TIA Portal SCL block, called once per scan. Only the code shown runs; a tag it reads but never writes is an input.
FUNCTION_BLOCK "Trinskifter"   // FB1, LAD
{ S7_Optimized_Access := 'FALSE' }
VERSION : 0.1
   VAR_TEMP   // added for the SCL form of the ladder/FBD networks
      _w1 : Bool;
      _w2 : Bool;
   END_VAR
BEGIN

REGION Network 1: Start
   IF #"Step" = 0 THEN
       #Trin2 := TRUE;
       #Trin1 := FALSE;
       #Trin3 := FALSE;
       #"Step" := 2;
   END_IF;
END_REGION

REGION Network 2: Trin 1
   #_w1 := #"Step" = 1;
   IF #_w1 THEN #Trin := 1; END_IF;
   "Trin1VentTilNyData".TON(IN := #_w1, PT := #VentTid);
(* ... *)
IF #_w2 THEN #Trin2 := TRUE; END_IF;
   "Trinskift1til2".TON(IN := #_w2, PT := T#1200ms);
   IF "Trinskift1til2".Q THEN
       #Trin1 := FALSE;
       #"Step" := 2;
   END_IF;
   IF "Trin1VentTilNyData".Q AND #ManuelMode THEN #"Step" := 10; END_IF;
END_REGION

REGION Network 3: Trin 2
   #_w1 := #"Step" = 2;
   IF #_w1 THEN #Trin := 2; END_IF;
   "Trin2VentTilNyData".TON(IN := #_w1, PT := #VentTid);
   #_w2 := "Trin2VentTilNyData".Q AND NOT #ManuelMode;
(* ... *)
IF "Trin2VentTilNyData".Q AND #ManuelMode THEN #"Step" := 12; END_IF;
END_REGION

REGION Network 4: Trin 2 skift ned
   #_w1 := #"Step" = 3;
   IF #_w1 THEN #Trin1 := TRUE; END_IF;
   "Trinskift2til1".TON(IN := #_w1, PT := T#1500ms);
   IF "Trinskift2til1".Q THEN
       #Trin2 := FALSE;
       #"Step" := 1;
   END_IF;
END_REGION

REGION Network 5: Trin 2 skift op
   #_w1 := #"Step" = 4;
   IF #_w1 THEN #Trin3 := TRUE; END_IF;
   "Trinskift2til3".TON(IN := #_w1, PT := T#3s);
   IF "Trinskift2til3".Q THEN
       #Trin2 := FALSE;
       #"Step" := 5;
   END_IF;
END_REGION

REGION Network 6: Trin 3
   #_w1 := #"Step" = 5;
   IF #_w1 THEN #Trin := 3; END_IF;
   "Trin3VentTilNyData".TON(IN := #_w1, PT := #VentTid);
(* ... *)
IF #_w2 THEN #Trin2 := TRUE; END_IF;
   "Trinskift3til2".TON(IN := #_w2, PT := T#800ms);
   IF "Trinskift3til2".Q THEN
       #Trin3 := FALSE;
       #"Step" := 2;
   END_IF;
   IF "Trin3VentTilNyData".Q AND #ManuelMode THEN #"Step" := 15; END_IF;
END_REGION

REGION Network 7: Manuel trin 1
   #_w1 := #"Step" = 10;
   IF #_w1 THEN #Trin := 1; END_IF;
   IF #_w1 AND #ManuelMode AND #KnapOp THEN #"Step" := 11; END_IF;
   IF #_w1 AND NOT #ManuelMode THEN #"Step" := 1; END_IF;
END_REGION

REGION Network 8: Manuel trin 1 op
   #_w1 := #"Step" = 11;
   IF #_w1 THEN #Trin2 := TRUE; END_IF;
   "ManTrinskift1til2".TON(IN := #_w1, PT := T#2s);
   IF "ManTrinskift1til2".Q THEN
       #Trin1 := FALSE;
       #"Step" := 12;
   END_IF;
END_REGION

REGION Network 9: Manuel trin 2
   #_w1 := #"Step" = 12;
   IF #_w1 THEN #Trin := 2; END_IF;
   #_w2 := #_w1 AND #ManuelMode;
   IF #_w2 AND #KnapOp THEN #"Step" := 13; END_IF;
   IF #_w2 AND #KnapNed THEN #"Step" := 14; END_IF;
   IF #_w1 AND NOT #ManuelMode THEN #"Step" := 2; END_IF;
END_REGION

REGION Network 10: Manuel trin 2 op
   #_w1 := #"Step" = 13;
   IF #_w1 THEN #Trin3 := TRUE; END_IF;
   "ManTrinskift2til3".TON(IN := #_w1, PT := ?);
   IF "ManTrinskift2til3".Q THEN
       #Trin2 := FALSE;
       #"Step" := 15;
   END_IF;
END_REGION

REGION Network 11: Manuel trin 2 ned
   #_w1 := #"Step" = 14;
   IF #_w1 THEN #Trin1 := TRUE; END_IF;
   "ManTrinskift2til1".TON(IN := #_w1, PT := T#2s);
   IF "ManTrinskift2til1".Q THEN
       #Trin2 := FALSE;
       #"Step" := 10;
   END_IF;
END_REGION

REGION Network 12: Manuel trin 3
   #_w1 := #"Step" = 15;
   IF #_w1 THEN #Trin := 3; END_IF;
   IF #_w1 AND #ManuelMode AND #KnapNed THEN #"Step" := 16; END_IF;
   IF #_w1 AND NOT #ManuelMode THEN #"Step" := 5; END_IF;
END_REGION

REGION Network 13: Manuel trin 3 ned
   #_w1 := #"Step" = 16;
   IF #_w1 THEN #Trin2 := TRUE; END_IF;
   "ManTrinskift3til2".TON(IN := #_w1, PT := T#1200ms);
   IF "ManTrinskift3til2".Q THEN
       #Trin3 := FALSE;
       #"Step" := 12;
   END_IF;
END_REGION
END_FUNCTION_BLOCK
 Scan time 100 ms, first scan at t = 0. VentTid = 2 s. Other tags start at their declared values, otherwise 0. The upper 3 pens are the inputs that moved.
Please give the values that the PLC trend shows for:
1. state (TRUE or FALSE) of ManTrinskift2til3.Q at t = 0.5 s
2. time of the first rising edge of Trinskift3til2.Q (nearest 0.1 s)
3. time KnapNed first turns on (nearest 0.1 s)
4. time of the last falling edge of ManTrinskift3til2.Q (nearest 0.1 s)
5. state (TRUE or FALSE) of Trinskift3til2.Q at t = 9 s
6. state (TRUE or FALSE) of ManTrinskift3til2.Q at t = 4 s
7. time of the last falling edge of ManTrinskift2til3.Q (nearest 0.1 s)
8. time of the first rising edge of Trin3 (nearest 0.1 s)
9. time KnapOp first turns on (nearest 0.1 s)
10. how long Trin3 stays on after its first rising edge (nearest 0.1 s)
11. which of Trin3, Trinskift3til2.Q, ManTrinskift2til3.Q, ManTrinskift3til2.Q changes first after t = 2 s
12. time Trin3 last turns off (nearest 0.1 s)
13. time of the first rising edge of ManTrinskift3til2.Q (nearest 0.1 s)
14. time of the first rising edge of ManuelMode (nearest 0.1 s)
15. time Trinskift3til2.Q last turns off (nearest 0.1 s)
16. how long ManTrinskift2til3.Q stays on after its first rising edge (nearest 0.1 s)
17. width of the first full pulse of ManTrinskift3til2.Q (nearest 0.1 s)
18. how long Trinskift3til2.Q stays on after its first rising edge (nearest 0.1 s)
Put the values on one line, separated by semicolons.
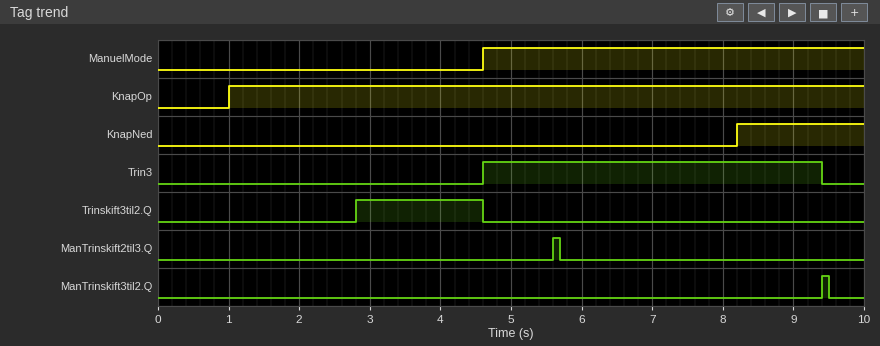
FALSE; 2.8 s; 8.2 s; 9.5 s; FALSE; FALSE; 5.7 s; 4.6 s; 1.0 s; 4.8 s; Trinskift3til2.Q; 9.4 s; 9.4 s; 4.6 s; 4.6 s; 0.1 s; 0.1 s; 1.8 s
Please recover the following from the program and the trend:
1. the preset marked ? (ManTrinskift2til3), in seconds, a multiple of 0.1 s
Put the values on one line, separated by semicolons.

1.0 s
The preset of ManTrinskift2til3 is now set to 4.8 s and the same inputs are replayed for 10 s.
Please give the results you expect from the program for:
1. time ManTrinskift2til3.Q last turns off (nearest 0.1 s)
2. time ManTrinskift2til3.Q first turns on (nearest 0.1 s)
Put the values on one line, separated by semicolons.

9.5 s; 9.4 s
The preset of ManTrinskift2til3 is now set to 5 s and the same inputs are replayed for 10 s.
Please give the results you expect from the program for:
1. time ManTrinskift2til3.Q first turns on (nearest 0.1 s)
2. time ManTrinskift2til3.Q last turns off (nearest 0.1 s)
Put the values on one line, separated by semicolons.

9.6 s; 9.7 s
